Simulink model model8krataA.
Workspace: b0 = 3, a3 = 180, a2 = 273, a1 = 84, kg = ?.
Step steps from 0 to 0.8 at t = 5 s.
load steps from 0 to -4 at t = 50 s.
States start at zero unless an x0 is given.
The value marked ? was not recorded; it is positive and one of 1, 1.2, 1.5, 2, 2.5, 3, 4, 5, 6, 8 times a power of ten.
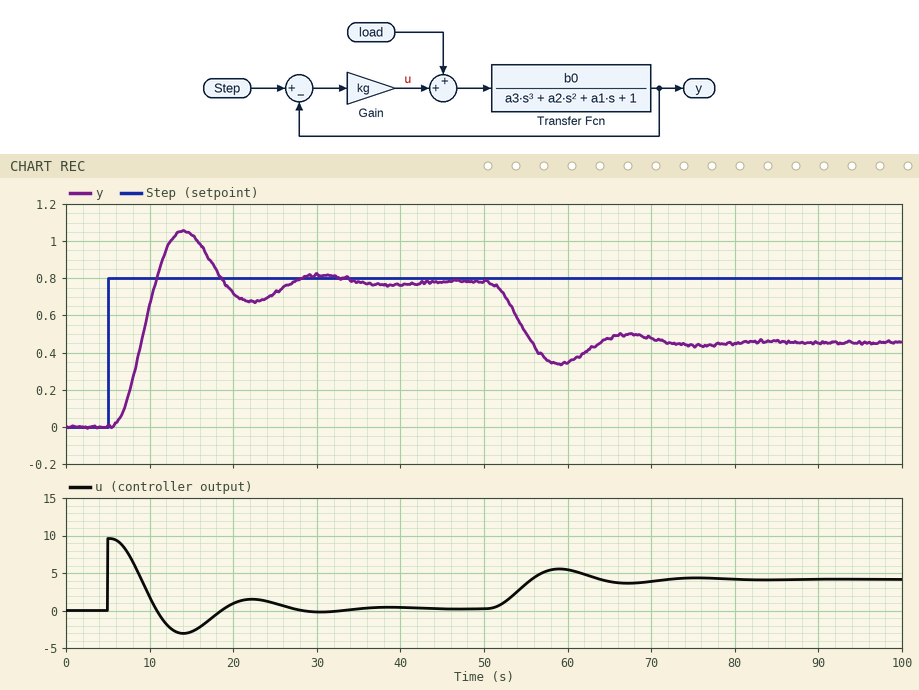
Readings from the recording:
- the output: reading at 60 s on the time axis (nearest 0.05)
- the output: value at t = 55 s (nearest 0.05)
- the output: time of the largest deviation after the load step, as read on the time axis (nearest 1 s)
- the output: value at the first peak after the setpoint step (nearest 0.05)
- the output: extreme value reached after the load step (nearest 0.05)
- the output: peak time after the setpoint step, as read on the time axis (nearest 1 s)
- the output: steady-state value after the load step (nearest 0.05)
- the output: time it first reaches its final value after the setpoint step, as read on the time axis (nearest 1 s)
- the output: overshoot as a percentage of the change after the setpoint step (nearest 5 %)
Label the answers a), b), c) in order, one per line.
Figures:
a) 0.35
b) 0.50
c) 59 s
d) 1.05
e) 0.35
f) 14 s
g) 0.45
h) 11 s
i) 35 %
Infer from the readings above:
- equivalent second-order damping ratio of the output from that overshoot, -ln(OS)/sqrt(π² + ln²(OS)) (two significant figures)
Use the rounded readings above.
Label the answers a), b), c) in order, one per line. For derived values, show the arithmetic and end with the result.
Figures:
a) ln(0.35) = -1.050; 1.050 / sqrt(9.870 + 1.102) = 0.32
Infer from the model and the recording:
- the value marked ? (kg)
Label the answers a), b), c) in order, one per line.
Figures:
a) 12
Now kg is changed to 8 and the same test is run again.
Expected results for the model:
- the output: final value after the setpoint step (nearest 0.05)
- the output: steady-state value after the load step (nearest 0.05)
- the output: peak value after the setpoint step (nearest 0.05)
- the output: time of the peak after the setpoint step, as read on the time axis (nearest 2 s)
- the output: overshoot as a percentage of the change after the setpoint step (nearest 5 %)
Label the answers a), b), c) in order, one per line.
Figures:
a) 0.75
b) 0.30
c) 0.95
d) 16 s
e) 20 %
